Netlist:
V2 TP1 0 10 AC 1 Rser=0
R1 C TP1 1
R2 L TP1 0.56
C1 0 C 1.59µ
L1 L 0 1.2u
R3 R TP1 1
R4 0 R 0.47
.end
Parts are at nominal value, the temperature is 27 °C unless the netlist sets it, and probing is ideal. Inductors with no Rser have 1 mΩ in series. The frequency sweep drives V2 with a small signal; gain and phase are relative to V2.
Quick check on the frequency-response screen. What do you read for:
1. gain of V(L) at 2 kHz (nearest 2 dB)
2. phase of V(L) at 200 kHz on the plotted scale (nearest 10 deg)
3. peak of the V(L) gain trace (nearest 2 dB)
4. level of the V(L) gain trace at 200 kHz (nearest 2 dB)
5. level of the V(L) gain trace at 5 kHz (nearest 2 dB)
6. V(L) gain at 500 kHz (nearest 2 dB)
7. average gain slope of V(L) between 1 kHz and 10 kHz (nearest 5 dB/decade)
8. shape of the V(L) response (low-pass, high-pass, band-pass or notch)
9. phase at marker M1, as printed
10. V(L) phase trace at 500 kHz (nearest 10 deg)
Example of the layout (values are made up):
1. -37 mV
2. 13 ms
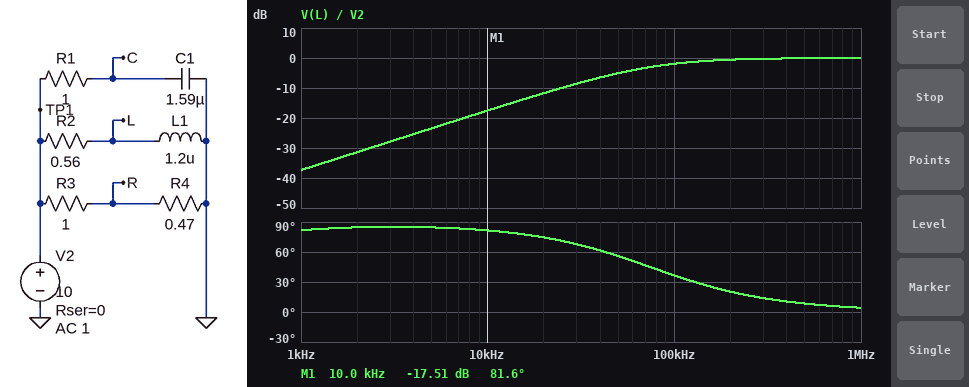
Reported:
1. -32 dB
2. 20 deg
3. 0 dB
4. 0 dB
5. -24 dB
6. 0 dB
7. 20 dB/decade
8. high-pass
9. 81.6 deg
10. 10 deg
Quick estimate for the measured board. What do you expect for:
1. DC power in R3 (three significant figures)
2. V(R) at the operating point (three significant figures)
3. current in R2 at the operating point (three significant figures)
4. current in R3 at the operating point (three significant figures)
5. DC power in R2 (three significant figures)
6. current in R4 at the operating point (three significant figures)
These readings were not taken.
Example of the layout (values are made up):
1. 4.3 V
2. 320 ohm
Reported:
1. 46.3 W
2. 3.20 V
3. 17.8 A
4. 6.80 A
5. 178 W
6. 6.80 A
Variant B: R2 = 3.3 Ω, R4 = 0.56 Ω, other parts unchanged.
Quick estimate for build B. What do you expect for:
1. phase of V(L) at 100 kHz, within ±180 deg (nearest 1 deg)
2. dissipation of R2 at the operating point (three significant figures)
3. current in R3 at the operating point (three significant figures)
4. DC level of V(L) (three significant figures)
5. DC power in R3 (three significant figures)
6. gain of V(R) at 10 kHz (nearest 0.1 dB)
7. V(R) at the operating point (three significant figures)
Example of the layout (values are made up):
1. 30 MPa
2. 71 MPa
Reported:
1. 77 deg
2. 30.3 W
3. 6.41 A
4. 3.03 mV
5. 41.1 W
6. -8.9 dB
7. 3.59 V
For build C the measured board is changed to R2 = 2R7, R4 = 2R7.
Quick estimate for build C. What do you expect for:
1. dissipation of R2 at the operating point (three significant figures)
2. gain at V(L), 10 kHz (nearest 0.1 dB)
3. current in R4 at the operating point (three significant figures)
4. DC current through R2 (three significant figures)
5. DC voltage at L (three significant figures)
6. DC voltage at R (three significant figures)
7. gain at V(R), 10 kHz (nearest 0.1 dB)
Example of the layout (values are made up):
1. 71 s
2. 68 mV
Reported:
1. 37.0 W
2. -31.1 dB
3. 2.70 A
4. 3.70 A
5. 3.70 mV
6. 7.30 V
7. -2.7 dB
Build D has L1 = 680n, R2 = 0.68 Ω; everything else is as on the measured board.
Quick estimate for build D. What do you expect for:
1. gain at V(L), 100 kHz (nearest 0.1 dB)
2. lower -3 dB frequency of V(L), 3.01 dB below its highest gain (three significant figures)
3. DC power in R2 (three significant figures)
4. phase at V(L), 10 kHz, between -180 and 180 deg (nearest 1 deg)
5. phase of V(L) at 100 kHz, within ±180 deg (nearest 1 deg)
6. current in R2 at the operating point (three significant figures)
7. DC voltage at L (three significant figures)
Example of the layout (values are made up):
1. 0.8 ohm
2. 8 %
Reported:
1. -5.5 dB
2. 159 kHz
3. 147 W
4. 85 deg
5. 58 deg
6. 14.7 A
7. 14.7 mV
